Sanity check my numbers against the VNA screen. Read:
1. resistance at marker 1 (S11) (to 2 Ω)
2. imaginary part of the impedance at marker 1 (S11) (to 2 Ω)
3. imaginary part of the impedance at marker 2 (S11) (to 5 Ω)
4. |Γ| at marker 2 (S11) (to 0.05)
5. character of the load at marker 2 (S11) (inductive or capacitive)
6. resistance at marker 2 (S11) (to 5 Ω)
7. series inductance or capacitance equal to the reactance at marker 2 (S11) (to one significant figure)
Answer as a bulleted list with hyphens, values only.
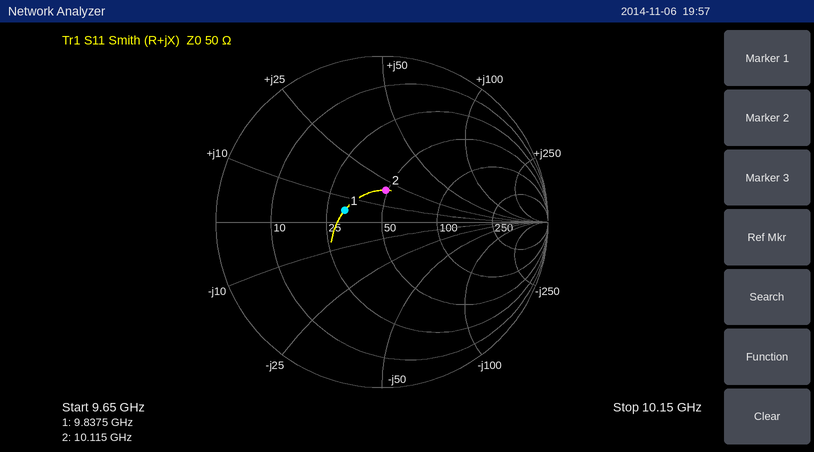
- 32 Ω
- +4 Ω
- +20 Ω
- 0.20
- inductive
- 50 Ω
- 300 pH
